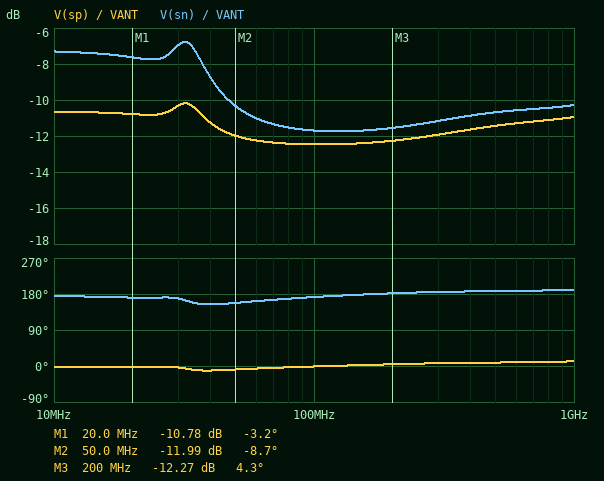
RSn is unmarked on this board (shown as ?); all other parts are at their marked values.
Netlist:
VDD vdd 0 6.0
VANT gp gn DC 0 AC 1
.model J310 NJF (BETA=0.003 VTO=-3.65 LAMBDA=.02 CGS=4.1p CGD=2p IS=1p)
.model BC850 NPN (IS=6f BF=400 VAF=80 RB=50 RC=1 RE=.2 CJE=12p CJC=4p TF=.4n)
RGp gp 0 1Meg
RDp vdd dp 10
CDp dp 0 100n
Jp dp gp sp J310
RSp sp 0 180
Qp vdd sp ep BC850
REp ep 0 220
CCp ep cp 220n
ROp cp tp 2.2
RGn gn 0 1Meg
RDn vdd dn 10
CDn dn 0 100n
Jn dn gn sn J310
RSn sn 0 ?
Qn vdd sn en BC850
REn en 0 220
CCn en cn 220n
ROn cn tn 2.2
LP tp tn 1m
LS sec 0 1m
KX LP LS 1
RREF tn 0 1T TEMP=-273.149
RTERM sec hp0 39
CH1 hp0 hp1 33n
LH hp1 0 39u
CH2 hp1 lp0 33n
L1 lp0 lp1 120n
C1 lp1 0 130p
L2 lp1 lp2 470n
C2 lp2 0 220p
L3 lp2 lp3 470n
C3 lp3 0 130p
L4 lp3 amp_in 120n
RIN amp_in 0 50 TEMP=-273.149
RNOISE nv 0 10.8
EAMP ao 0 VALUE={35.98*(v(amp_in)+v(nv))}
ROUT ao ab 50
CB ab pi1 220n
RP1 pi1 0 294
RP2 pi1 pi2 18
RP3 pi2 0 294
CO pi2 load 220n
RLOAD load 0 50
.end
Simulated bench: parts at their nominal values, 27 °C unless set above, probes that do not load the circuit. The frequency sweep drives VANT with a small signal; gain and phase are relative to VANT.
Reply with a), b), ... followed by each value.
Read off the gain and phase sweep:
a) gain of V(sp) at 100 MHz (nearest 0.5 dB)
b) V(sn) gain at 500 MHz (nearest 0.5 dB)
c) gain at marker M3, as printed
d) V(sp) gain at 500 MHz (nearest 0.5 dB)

a) -12.5 dB
b) -10.5 dB
c) -12.27 dB
d) -11.5 dB
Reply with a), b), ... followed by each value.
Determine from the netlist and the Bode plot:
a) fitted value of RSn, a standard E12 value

a) 470 Ω
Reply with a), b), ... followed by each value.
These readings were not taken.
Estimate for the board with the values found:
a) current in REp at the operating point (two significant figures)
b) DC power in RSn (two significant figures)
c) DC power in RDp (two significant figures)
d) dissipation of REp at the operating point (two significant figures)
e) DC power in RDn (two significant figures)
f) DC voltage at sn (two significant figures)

a) 5.2 mA
b) 12 mW
c) 1.1 mW
d) 6.0 mW
e) 260 µW
f) 2.4 V
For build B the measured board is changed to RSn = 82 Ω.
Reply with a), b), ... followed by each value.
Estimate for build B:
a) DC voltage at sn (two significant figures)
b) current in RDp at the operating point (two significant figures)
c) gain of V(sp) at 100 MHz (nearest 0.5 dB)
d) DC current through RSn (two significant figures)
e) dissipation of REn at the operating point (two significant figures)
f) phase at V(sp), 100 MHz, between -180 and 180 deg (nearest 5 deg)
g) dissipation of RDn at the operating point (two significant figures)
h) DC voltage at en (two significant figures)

a) 1.4 V
b) 10 mA
c) -11.0 dB
d) 17 mA
e) 2.1 mW
f) -5 deg
g) 2.8 mW
h) 680 mV
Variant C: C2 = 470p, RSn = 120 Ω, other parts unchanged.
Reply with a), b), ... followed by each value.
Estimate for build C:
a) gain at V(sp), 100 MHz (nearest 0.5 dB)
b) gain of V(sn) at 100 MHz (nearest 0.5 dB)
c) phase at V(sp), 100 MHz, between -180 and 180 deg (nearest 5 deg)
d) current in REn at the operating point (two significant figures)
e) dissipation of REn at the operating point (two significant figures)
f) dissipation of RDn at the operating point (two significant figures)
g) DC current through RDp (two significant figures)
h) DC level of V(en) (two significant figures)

a) -11.5 dB
b) -13.0 dB
c) -5 deg
d) 4.1 mA
e) 3.8 mW
f) 1.8 mW
g) 10 mA
h) 910 mV
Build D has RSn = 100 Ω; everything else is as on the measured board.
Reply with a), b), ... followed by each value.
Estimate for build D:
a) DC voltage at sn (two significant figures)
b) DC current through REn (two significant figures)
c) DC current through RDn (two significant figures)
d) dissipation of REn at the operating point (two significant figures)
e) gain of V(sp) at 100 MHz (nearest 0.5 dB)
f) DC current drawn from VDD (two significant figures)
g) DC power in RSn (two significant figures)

a) 1.5 V
b) 3.6 mA
c) 15 mA
d) 2.9 mW
e) -11.5 dB
f) 34 mA
g) 23 mW
